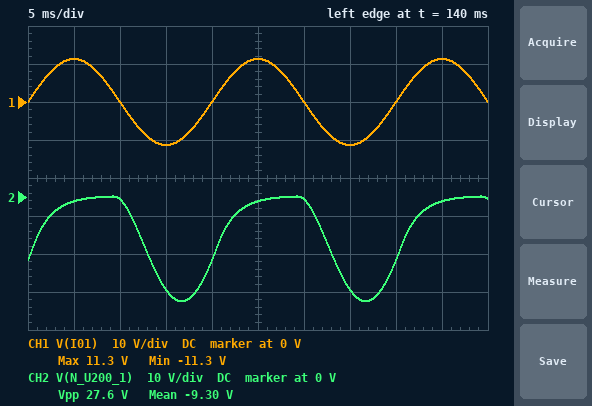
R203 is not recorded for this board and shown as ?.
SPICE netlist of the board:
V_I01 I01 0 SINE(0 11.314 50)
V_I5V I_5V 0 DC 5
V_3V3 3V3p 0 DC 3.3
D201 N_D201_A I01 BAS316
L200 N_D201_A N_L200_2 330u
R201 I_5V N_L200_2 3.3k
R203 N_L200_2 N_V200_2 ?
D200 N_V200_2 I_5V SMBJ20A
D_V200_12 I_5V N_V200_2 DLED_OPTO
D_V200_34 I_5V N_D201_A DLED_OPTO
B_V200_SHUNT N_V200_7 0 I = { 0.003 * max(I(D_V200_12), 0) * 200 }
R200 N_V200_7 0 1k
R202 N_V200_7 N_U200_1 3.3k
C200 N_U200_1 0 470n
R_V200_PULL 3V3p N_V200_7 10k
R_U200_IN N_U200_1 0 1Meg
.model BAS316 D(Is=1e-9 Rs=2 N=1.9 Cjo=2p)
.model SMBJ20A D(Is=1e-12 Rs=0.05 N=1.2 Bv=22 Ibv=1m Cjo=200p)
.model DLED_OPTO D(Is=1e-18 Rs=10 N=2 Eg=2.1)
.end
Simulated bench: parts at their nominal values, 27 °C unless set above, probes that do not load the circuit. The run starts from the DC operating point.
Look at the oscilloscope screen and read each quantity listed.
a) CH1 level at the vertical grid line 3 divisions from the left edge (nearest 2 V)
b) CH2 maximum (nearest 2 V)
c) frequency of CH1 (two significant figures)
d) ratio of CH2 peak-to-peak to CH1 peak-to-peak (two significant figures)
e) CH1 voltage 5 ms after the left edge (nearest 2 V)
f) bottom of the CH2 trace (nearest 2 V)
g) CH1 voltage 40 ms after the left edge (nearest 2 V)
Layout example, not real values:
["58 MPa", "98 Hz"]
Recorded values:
["-12 V", "0 V", "50 Hz", "1.2", "12 V", "-28 V", "0 V"]
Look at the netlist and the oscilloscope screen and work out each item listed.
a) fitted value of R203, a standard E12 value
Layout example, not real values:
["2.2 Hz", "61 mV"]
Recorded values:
["180 Ω"]
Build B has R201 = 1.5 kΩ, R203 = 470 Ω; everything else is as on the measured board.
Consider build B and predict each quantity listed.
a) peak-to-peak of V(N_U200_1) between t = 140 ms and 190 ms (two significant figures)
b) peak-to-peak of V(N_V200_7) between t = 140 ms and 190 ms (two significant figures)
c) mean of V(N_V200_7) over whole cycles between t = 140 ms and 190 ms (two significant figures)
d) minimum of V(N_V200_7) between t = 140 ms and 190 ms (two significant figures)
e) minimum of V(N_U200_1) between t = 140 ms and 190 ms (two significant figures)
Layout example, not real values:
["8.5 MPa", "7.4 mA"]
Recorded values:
["11 V", "12 V", "-4.2 V", "-12 V", "-11 V"]
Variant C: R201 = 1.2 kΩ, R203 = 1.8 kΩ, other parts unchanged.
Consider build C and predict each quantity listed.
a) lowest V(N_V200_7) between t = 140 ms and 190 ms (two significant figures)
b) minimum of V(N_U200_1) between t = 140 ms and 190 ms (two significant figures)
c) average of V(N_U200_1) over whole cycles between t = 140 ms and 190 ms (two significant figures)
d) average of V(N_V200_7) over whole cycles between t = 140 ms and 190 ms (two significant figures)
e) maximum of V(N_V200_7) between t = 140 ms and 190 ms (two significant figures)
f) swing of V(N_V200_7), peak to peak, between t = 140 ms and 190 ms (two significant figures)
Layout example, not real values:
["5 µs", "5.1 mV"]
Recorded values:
["-2.9 V", "-2.7 V", "-890 mV", "-900 mV", "300 mV", "3.2 V"]
